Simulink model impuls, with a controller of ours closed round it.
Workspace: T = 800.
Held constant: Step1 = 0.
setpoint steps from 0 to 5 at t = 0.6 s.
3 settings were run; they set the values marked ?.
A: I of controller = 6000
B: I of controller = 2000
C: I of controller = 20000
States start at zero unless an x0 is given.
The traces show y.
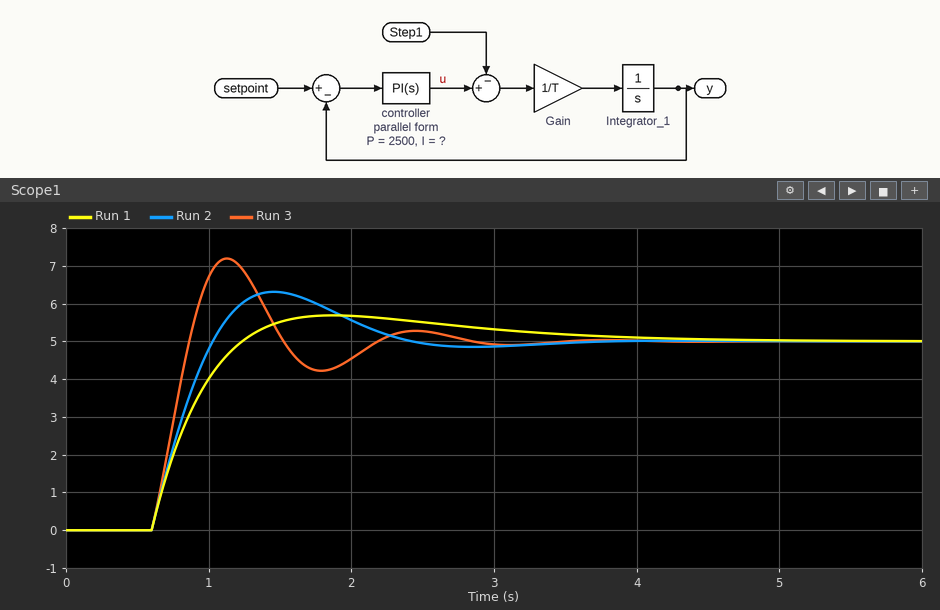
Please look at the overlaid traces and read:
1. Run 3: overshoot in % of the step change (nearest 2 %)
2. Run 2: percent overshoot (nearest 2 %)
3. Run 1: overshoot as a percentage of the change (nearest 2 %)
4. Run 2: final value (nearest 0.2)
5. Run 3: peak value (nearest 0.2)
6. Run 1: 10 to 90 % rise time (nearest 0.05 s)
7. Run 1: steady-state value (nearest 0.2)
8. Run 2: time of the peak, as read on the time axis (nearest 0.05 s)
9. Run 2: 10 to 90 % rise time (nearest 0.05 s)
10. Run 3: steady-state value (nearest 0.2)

44 %
26 %
14 %
5.0
7.2
0.45 s
5.0
1.45 s
0.35 s
5.0
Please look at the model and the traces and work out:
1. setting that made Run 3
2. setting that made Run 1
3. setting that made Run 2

C
B
A
